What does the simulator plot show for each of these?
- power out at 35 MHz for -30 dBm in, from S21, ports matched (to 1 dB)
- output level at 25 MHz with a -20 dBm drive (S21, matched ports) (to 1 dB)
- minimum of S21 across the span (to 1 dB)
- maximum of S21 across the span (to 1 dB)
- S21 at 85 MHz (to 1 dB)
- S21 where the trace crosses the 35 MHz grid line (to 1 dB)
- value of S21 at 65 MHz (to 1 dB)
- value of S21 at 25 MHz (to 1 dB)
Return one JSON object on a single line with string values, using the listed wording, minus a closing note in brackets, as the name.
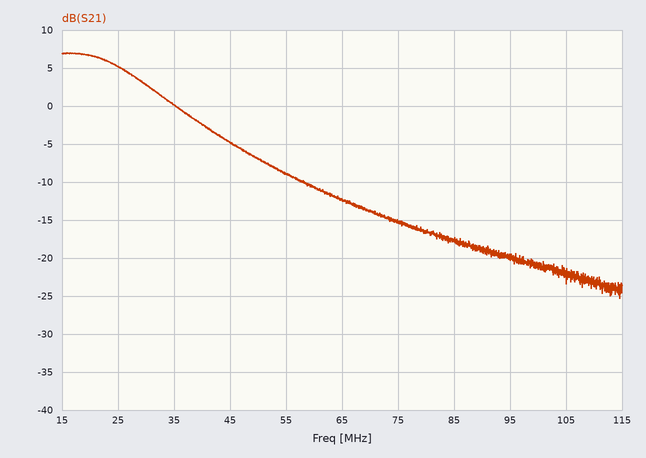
{"power out at 35 MHz for -30 dBm in, from S21, ports matched": "-30 dBm", "output level at 25 MHz with a -20 dBm drive (S21, matched ports)": "-15 dBm", "minimum of S21 across the span": "-25 dB", "maximum of S21 across the span": "7 dB", "S21 at 85 MHz": "-18 dB", "S21 where the trace crosses the 35 MHz grid line": "0 dB", "value of S21 at 65 MHz": "-12 dB", "value of S21 at 25 MHz": "5 dB"}
